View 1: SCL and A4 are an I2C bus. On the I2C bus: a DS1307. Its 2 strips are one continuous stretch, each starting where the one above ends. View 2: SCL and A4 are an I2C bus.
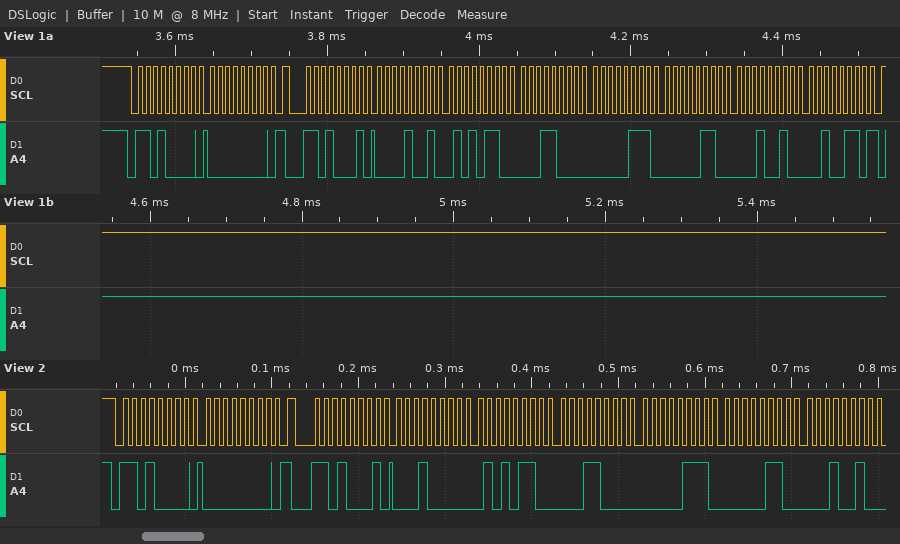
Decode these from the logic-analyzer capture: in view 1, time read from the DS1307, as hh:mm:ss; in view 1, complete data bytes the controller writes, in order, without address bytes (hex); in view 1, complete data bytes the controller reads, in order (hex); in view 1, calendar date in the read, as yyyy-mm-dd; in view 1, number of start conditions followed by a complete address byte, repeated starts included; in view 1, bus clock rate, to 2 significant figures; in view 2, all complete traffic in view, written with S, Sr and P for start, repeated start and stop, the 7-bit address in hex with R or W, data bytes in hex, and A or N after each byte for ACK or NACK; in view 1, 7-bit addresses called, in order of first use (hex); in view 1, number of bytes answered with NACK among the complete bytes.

18:56:09
00
09 56 18 07 06 12 26
2026-12-06
2
100 kHz
S 68W A 00 A Sr 68R A 10 A 56 A 18 A 07 A 06 A 12 A
0x68
1
